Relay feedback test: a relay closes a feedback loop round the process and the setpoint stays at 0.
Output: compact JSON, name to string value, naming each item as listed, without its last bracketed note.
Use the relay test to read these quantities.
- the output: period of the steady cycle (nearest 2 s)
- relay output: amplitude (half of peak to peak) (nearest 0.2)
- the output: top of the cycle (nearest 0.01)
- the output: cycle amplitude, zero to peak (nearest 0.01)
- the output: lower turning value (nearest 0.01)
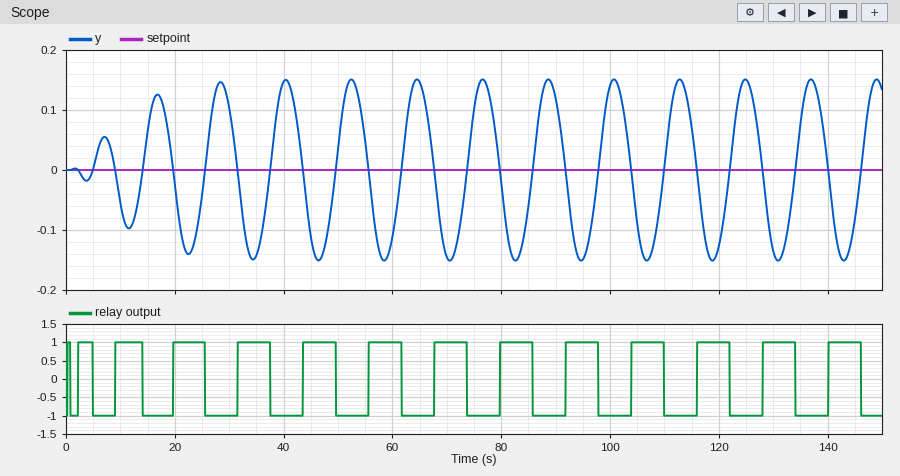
{"the output: period of the steady cycle": "12 s", "relay output: amplitude (half of peak to peak)": "1.0", "the output: top of the cycle": "0.15", "the output: cycle amplitude, zero to peak": "0.15", "the output: lower turning value": "-0.15"}
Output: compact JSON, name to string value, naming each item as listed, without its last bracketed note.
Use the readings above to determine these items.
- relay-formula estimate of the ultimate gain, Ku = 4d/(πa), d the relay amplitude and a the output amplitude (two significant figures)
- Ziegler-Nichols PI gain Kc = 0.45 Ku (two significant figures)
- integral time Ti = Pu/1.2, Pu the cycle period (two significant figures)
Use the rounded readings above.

{"relay-formula estimate of the ultimate gain, Ku = 4d/(πa), d the relay amplitude and a the output amplitude": "8.5", "Ziegler-Nichols PI gain Kc = 0.45 Ku": "3.8", "integral time Ti = Pu/1.2, Pu the cycle period": "10 s"}
